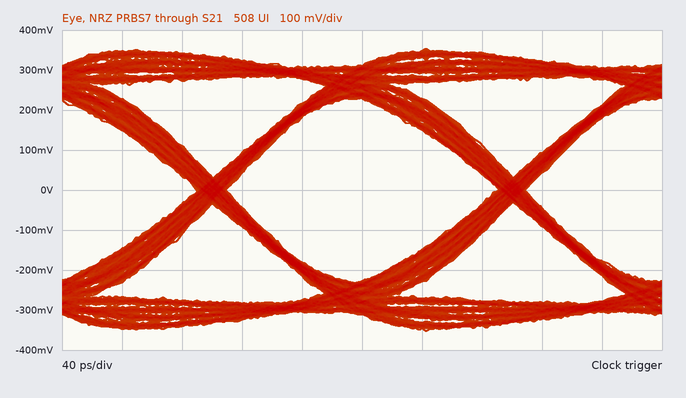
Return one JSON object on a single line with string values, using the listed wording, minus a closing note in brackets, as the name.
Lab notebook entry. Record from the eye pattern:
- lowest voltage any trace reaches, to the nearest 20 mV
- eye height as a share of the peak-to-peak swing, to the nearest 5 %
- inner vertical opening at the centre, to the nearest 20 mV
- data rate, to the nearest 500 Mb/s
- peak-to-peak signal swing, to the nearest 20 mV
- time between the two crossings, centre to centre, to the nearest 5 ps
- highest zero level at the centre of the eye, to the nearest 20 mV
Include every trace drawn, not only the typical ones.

{"lowest voltage any trace reaches, to the nearest 20 mV": "-360 mV", "eye height as a share of the peak-to-peak swing, to the nearest 5 %": "65 %", "inner vertical opening at the centre, to the nearest 20 mV": "460 mV", "data rate, to the nearest 500 Mb/s": "5.0 Gb/s", "peak-to-peak signal swing, to the nearest 20 mV": "700 mV", "time between the two crossings, centre to centre, to the nearest 5 ps": "200 ps", "highest zero level at the centre of the eye, to the nearest 20 mV": "-220 mV"}
